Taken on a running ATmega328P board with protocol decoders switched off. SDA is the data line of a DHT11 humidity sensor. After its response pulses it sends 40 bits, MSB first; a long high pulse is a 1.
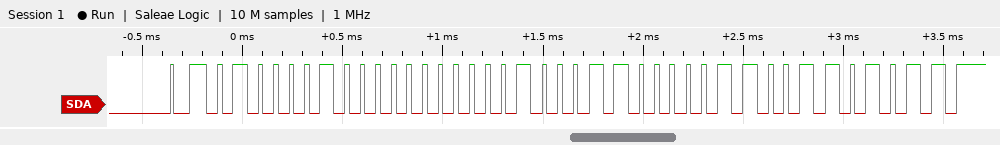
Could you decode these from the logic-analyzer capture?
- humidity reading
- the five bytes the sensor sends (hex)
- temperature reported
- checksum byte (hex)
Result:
66 %
42 00 23 06 6B
35.6 °C
0x6B
